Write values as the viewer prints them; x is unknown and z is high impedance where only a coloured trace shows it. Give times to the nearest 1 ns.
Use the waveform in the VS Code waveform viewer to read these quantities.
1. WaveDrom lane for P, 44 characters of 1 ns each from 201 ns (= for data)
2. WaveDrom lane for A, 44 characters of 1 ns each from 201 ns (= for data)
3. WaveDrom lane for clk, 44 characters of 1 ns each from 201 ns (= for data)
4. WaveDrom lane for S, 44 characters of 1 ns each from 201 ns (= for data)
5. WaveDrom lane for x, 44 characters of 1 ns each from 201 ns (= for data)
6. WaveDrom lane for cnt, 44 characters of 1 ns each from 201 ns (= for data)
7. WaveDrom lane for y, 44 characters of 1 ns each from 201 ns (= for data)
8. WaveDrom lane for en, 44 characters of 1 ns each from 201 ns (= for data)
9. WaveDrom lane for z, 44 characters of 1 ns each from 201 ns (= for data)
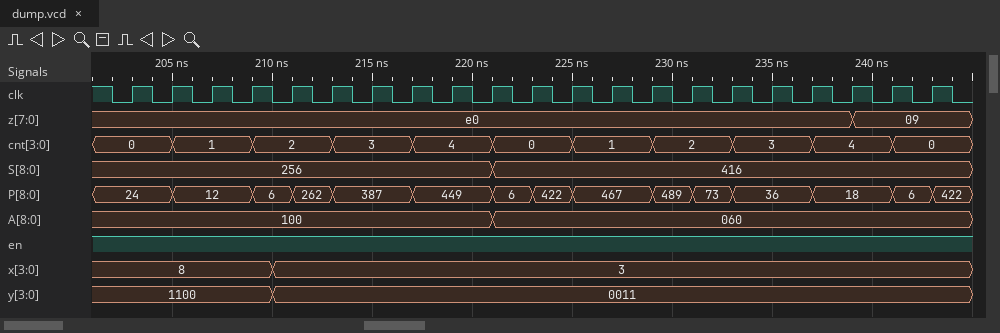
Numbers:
{name: 'P', wave: '=...=...=.=.=...=...=.=.=...=.=.=...=...=.=.', data: '24 12 6 262 387 449 6 422 467 489 73 36 18 6 422'}
{name: 'A', wave: '=...................=.......................', data: '100 060'}
{name: 'clk', wave: '10101010101010101010101010101010101010101010'}
{name: 'S', wave: '=...................=.......................', data: '256 416'}
{name: 'x', wave: '=........=..................................', data: '8 3'}
{name: 'cnt', wave: '=...=...=...=...=...=...=...=...=...=...=...', data: '0 1 2 3 4 0 1 2 3 4 0'}
{name: 'y', wave: '=........=..................................', data: '1100 0011'}
{name: 'en', wave: '1...........................................'}
{name: 'z', wave: '=.....................................=.....', data: 'e0 09'}
